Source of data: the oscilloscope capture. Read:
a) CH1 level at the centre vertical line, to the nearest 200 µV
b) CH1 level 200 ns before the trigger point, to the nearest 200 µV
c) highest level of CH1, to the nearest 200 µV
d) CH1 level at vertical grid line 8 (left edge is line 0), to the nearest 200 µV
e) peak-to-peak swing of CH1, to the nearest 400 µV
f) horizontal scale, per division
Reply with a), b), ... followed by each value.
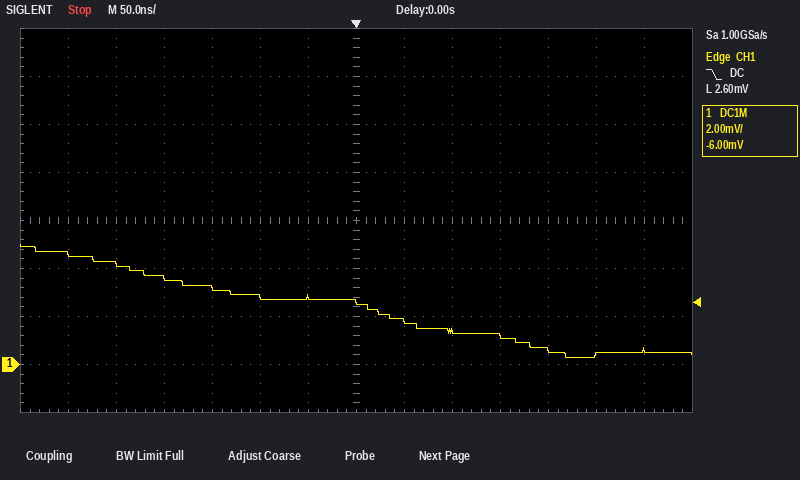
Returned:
a) 2.6 mV
b) 3.6 mV
c) 5.0 mV
d) 1.8 mV
e) 4.8 mV
f) 50 ns
